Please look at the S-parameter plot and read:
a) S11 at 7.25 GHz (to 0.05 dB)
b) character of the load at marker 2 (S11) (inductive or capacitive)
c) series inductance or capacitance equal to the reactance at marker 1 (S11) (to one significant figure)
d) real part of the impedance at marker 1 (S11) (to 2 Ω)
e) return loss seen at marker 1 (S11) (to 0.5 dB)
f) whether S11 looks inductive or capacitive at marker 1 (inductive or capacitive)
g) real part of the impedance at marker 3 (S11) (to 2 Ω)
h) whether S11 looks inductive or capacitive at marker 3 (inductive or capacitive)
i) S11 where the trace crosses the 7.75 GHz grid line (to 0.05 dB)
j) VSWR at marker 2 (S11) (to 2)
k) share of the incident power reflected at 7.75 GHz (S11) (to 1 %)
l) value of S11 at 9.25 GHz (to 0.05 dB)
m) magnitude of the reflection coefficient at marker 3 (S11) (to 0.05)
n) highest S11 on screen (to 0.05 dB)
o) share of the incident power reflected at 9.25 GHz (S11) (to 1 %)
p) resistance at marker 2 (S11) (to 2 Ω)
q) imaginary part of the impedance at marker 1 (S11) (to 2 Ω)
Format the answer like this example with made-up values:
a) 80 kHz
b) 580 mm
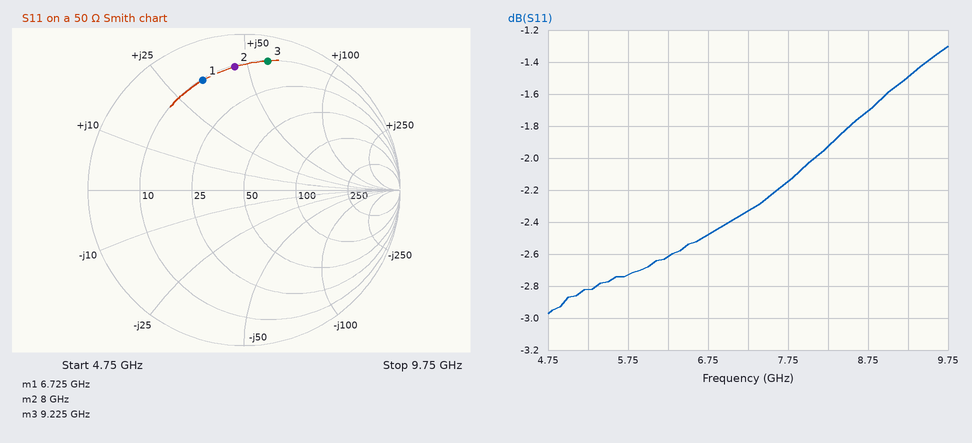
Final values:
a) -2.35 dB
b) inductive
c) 800 pH
d) 10 Ω
e) 2.5 dB
f) inductive
g) 10 Ω
h) inductive
i) -2.15 dB
j) 8
k) 61 %
l) -1.50 dB
m) 0.85
n) -1.30 dB
o) 71 %
p) 10 Ω
q) +34 Ω
